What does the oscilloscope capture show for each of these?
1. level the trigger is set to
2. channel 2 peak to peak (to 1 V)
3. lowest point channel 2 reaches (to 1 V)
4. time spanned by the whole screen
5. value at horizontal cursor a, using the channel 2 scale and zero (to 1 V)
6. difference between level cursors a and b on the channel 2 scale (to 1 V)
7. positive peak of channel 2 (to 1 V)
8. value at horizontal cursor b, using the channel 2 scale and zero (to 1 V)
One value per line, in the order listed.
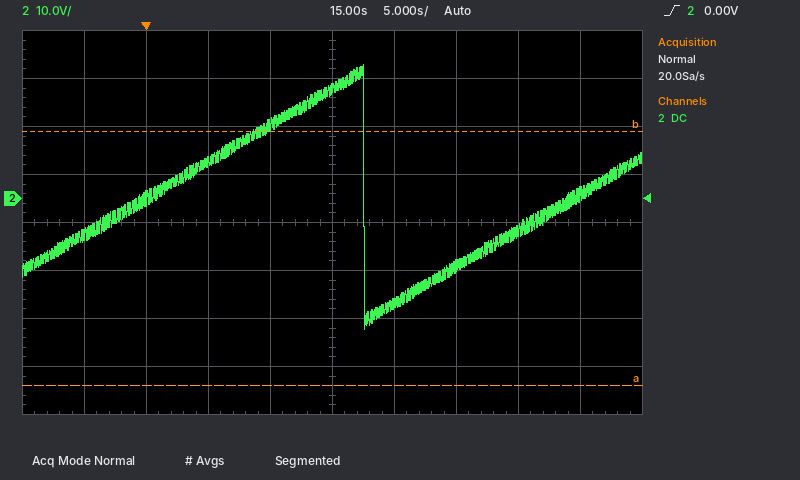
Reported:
0.00 V
55 V
-27 V
50 s
-39 V
53 V
28 V
14 V
